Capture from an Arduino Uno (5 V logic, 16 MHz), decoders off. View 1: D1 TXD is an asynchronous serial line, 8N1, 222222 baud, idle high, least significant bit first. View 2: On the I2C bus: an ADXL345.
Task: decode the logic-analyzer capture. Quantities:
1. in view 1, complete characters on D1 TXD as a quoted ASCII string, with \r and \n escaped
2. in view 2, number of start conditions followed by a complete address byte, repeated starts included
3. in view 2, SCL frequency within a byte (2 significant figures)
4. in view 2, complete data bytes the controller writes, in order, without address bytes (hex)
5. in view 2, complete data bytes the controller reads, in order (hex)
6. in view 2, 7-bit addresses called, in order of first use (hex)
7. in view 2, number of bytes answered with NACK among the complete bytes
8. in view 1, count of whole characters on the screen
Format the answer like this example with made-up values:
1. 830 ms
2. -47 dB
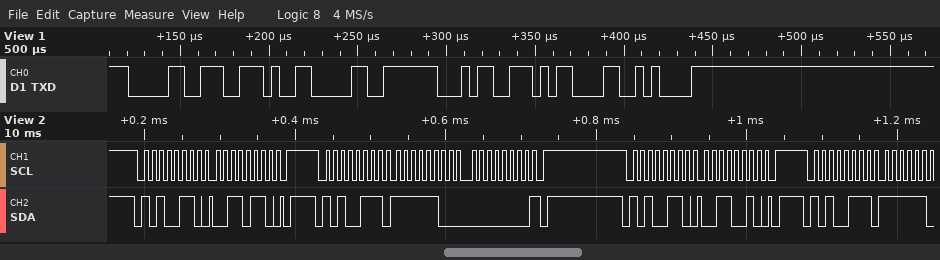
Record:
1. "0.04\r\n"
2. 4
3. 100 kHz
4. 36 32
5. FC 00
6. 0x53
7. 1
8. 6
